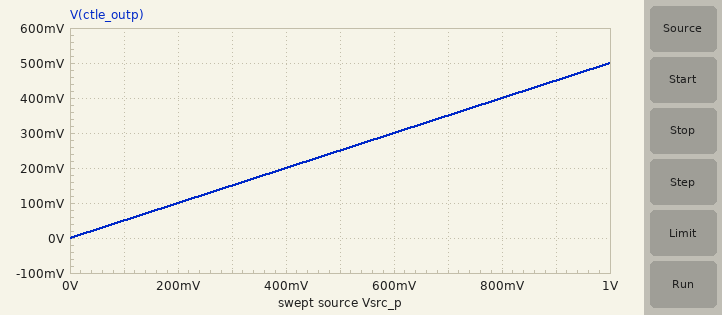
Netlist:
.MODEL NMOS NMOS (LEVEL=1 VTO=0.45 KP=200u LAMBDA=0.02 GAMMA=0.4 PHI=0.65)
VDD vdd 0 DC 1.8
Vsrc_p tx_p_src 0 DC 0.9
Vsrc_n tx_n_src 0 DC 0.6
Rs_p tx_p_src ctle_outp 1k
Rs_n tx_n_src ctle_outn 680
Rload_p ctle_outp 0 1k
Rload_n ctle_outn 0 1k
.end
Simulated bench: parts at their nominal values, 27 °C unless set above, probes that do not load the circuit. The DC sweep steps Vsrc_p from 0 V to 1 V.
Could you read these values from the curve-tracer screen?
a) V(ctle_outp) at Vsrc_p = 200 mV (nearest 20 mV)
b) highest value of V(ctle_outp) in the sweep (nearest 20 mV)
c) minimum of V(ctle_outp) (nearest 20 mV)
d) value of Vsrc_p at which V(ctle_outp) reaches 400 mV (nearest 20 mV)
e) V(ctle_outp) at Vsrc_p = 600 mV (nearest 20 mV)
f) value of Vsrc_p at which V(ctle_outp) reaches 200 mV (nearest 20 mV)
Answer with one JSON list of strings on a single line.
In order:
["100 mV", "500 mV", "0 V", "800 mV", "300 mV", "400 mV"]
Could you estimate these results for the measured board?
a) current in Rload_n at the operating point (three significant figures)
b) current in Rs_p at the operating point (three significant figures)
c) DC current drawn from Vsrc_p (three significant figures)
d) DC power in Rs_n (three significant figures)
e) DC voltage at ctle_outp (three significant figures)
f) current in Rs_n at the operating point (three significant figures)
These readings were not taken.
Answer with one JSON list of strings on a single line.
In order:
["357 µA", "450 µA", "450 µA", "86.7 µW", "450 mV", "357 µA"]
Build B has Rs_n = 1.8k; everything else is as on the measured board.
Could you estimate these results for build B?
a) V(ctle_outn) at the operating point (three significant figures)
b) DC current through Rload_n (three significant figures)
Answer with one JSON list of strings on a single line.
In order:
["214 mV", "214 µA"]
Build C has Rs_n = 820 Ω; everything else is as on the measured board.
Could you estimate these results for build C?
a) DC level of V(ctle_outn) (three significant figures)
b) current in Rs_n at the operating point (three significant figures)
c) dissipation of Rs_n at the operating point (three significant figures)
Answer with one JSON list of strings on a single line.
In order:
["330 mV", "330 µA", "89.1 µW"]
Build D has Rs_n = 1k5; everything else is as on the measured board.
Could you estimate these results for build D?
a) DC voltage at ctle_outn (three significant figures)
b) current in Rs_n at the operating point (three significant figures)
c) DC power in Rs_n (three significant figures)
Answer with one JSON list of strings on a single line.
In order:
["240 mV", "240 µA", "86.4 µW"]
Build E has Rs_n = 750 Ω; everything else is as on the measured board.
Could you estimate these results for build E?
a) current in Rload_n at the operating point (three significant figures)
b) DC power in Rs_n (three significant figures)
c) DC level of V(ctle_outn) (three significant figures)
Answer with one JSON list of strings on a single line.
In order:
["343 µA", "88.2 µW", "343 mV"]
